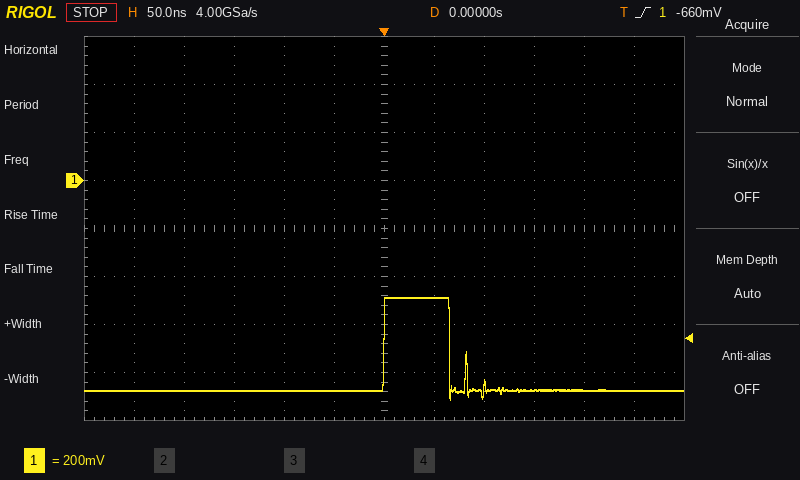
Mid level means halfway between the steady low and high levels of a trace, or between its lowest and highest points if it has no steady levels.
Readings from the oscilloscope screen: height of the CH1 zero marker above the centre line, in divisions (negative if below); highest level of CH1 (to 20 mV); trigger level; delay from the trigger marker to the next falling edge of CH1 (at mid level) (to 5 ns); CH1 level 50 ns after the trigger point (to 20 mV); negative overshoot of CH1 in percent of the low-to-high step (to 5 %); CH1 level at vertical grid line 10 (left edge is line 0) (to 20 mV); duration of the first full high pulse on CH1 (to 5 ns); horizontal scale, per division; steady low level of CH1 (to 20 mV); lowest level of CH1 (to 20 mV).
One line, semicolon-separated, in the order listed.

+1.0 div; -480 mV; -660 mV; 65 ns; -480 mV; 10 %; -880 mV; 65 ns; 50 ns; -880 mV; -920 mV
